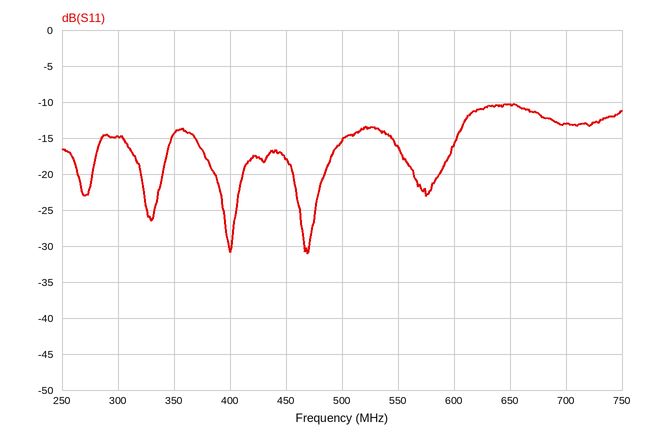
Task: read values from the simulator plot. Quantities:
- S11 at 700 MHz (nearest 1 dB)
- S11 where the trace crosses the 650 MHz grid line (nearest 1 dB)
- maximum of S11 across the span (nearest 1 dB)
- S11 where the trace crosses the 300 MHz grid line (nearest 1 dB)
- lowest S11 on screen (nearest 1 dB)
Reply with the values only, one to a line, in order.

-13 dB
-10 dB
-10 dB
-15 dB
-31 dB
